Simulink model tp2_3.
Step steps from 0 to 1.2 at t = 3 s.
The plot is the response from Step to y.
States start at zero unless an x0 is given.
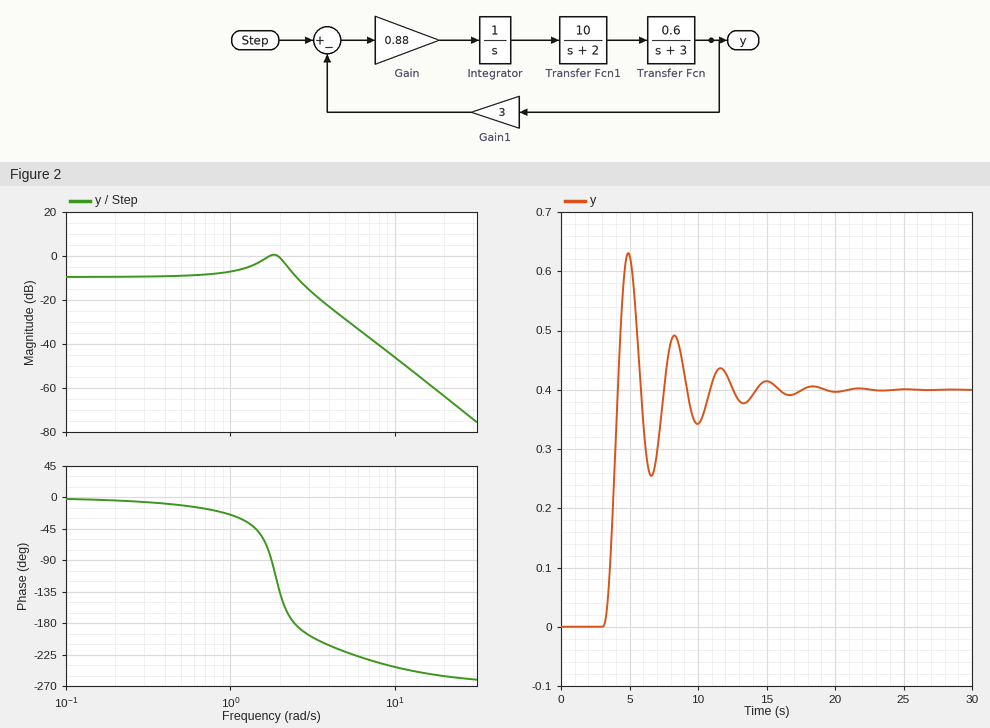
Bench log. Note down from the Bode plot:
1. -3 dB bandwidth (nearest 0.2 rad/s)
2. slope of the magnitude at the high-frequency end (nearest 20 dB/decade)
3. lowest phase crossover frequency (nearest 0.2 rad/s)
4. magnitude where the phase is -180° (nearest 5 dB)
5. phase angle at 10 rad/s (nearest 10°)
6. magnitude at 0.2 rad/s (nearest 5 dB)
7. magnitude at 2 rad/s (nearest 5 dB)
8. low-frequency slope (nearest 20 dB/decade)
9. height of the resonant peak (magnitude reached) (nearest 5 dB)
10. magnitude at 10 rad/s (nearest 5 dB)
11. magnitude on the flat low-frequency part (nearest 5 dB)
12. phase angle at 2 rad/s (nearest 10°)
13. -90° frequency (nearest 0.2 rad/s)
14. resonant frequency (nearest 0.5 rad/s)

2.8 rad/s
-60 dB/decade
2.4 rad/s
-10 dB
-240°
-10 dB
0 dB
0 dB/decade
0 dB
-45 dB
-10 dB
-140°
1.8 rad/s
2.0 rad/s
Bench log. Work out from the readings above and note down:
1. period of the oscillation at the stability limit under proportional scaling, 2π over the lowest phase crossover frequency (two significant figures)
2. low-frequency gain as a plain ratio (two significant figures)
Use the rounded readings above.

2.6 s
0.32
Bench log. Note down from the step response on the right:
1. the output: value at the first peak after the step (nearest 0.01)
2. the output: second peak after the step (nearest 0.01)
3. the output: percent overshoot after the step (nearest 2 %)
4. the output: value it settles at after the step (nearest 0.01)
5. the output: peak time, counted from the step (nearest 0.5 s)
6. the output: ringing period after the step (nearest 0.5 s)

0.63
0.49
58 %
0.40
2.0 s
3.5 s
